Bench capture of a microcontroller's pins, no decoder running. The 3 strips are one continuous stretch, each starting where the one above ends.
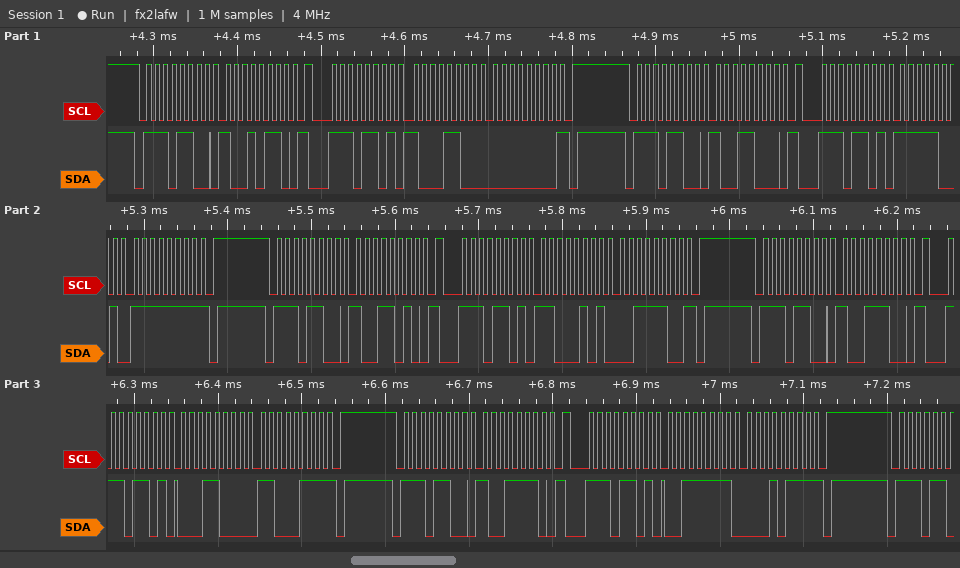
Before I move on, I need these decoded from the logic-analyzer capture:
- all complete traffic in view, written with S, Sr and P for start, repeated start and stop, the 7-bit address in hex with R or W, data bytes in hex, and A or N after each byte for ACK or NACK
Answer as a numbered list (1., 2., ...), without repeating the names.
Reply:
1. S 76W A 96 A Sr 76R A 8C A 00 N P S 76W A 98 A Sr 76R A F9 A FF N P S 76W A 9A A Sr 76R A C5 A 3C N P S 76W A 9C A Sr 76R A 18 A C7 N P S 76W A 9E A Sr 76R A 3F A 17 N P
